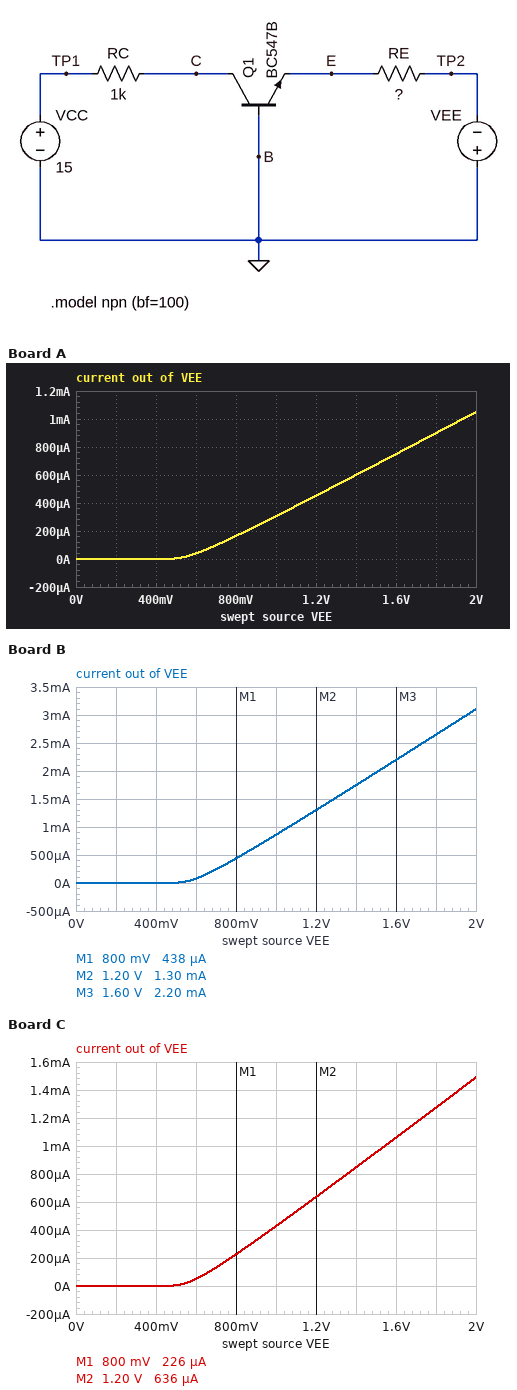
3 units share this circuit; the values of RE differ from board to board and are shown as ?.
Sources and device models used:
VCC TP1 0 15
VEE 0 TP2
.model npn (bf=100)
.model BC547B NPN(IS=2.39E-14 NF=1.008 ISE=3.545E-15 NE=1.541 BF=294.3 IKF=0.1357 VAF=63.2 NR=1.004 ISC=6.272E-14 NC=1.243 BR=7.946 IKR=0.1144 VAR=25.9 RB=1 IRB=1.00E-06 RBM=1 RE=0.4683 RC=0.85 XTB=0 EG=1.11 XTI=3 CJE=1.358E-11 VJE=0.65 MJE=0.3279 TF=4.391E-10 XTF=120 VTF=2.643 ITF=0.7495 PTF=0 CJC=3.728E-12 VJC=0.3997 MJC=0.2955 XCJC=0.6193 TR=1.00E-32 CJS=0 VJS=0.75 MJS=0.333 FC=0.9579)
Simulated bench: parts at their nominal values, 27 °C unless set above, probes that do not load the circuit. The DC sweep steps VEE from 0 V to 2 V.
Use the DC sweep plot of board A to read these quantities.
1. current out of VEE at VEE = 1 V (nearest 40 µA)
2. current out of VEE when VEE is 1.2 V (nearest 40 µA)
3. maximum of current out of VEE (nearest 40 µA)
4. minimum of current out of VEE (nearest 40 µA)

320 µA
440 µA
1.04 mA
0 A
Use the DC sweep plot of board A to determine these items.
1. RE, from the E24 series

1.3 kΩ
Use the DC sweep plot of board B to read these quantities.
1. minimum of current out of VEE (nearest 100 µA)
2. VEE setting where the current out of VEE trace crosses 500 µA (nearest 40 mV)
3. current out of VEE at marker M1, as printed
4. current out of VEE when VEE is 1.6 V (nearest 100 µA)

0 A
840 mV
438 µA
2.2 mA
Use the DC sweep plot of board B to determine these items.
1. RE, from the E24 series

430 Ω
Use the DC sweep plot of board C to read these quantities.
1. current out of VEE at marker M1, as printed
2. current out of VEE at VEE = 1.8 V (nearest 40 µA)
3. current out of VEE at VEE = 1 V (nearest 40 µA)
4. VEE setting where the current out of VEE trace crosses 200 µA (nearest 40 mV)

226 µA
1.28 mA
440 µA
760 mV
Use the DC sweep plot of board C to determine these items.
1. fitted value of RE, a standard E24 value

910 Ω
